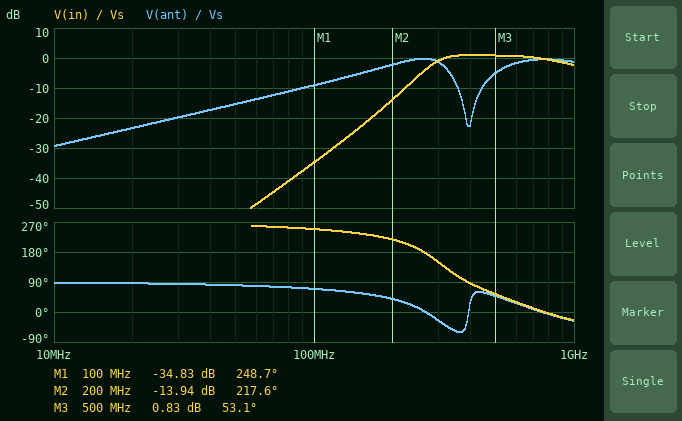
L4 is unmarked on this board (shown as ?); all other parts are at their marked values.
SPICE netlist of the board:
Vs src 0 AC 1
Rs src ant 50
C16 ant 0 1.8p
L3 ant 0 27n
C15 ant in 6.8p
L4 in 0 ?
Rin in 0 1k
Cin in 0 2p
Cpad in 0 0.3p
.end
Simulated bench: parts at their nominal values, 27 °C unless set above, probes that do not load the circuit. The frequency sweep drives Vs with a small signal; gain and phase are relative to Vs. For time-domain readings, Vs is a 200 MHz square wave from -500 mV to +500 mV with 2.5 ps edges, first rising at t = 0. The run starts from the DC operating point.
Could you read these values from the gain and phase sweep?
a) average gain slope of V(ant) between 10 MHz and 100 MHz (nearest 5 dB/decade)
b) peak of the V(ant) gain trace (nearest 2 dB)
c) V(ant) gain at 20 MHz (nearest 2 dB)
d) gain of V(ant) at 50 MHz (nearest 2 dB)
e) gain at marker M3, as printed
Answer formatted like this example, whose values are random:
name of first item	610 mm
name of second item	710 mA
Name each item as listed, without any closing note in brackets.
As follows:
average gain slope of V(ant) between 10 MHz and 100 MHz	20 dB/decade
peak of the V(ant) gain trace	0 dB
V(ant) gain at 20 MHz	-24 dB
gain of V(ant) at 50 MHz	-16 dB
gain at marker M3, as printed	0.83 dB
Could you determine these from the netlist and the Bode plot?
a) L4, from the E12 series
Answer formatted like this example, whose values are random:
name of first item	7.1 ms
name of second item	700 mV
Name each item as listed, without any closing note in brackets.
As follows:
L4, from the E12 series	18 nH
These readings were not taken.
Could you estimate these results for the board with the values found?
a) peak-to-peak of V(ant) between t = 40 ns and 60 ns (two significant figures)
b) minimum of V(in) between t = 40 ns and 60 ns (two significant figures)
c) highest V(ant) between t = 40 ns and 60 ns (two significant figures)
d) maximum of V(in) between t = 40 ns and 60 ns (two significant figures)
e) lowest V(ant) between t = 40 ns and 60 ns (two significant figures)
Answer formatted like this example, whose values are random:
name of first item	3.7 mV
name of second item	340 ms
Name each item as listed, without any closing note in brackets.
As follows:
peak-to-peak of V(ant) between t = 40 ns and 60 ns	1.6 V
minimum of V(in) between t = 40 ns and 60 ns	-340 mV
highest V(ant) between t = 40 ns and 60 ns	780 mV
maximum of V(in) between t = 40 ns and 60 ns	340 mV
lowest V(ant) between t = 40 ns and 60 ns	-780 mV
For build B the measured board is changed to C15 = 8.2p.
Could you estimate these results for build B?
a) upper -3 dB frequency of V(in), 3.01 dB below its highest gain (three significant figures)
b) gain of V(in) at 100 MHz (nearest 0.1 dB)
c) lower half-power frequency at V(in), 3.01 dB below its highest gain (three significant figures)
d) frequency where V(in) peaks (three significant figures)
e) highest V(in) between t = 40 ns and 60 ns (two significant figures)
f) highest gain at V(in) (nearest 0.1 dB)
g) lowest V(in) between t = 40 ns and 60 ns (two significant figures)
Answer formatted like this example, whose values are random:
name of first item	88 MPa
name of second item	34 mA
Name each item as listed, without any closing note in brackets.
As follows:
upper -3 dB frequency of V(in), 3.01 dB below its highest gain	1.05 GHz
gain of V(in) at 100 MHz	-33.0 dB
lower half-power frequency at V(in), 3.01 dB below its highest gain	258 MHz
frequency where V(in) peaks	582 MHz
highest V(in) between t = 40 ns and 60 ns	380 mV
highest gain at V(in)	0.3 dB
lowest V(in) between t = 40 ns and 60 ns	-380 mV
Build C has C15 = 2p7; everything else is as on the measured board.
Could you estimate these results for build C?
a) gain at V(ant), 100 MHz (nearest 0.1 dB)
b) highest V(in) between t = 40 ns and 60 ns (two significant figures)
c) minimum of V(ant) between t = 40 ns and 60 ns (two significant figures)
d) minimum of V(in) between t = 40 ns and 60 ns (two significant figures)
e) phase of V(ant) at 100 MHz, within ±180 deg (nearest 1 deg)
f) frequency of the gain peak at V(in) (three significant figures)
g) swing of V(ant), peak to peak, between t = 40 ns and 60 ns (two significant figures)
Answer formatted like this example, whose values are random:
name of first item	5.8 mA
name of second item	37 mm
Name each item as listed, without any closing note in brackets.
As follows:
gain at V(ant), 100 MHz	-9.5 dB
highest V(in) between t = 40 ns and 60 ns	440 mV
minimum of V(ant) between t = 40 ns and 60 ns	-720 mV
minimum of V(in) between t = 40 ns and 60 ns	-440 mV
phase of V(ant) at 100 MHz, within ±180 deg	70 deg
frequency of the gain peak at V(in)	538 MHz
swing of V(ant), peak to peak, between t = 40 ns and 60 ns	1.4 V
